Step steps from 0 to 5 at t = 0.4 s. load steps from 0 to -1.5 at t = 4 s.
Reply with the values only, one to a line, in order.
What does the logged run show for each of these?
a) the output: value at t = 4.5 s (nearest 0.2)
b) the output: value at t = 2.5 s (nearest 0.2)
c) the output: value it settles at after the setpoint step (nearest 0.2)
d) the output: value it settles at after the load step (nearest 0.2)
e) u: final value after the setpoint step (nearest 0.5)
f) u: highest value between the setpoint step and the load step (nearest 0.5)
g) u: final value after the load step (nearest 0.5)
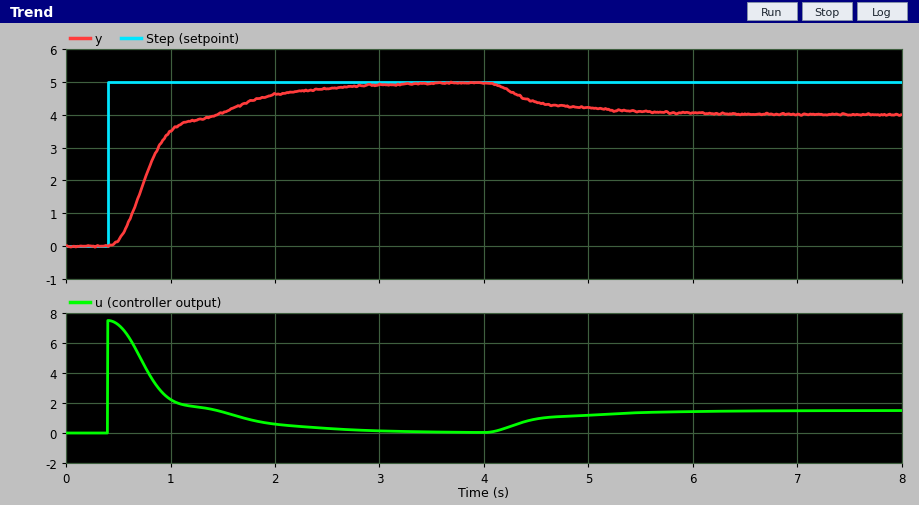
4.4
4.8
5.0
4.0
0.0
7.5
1.5
